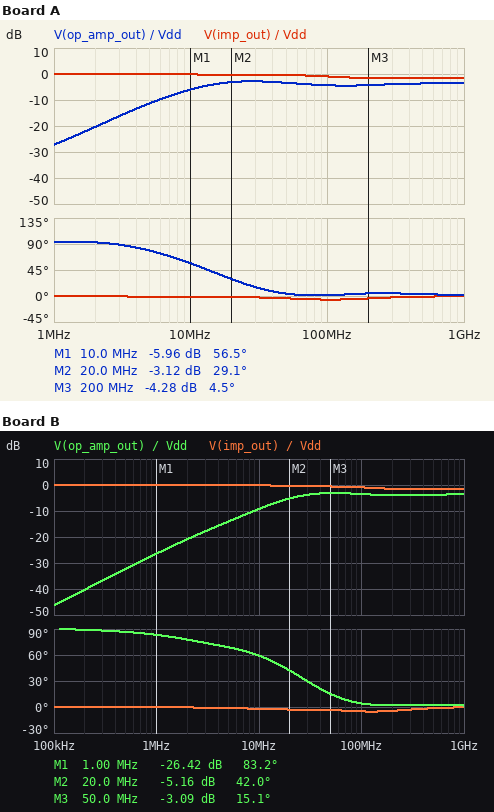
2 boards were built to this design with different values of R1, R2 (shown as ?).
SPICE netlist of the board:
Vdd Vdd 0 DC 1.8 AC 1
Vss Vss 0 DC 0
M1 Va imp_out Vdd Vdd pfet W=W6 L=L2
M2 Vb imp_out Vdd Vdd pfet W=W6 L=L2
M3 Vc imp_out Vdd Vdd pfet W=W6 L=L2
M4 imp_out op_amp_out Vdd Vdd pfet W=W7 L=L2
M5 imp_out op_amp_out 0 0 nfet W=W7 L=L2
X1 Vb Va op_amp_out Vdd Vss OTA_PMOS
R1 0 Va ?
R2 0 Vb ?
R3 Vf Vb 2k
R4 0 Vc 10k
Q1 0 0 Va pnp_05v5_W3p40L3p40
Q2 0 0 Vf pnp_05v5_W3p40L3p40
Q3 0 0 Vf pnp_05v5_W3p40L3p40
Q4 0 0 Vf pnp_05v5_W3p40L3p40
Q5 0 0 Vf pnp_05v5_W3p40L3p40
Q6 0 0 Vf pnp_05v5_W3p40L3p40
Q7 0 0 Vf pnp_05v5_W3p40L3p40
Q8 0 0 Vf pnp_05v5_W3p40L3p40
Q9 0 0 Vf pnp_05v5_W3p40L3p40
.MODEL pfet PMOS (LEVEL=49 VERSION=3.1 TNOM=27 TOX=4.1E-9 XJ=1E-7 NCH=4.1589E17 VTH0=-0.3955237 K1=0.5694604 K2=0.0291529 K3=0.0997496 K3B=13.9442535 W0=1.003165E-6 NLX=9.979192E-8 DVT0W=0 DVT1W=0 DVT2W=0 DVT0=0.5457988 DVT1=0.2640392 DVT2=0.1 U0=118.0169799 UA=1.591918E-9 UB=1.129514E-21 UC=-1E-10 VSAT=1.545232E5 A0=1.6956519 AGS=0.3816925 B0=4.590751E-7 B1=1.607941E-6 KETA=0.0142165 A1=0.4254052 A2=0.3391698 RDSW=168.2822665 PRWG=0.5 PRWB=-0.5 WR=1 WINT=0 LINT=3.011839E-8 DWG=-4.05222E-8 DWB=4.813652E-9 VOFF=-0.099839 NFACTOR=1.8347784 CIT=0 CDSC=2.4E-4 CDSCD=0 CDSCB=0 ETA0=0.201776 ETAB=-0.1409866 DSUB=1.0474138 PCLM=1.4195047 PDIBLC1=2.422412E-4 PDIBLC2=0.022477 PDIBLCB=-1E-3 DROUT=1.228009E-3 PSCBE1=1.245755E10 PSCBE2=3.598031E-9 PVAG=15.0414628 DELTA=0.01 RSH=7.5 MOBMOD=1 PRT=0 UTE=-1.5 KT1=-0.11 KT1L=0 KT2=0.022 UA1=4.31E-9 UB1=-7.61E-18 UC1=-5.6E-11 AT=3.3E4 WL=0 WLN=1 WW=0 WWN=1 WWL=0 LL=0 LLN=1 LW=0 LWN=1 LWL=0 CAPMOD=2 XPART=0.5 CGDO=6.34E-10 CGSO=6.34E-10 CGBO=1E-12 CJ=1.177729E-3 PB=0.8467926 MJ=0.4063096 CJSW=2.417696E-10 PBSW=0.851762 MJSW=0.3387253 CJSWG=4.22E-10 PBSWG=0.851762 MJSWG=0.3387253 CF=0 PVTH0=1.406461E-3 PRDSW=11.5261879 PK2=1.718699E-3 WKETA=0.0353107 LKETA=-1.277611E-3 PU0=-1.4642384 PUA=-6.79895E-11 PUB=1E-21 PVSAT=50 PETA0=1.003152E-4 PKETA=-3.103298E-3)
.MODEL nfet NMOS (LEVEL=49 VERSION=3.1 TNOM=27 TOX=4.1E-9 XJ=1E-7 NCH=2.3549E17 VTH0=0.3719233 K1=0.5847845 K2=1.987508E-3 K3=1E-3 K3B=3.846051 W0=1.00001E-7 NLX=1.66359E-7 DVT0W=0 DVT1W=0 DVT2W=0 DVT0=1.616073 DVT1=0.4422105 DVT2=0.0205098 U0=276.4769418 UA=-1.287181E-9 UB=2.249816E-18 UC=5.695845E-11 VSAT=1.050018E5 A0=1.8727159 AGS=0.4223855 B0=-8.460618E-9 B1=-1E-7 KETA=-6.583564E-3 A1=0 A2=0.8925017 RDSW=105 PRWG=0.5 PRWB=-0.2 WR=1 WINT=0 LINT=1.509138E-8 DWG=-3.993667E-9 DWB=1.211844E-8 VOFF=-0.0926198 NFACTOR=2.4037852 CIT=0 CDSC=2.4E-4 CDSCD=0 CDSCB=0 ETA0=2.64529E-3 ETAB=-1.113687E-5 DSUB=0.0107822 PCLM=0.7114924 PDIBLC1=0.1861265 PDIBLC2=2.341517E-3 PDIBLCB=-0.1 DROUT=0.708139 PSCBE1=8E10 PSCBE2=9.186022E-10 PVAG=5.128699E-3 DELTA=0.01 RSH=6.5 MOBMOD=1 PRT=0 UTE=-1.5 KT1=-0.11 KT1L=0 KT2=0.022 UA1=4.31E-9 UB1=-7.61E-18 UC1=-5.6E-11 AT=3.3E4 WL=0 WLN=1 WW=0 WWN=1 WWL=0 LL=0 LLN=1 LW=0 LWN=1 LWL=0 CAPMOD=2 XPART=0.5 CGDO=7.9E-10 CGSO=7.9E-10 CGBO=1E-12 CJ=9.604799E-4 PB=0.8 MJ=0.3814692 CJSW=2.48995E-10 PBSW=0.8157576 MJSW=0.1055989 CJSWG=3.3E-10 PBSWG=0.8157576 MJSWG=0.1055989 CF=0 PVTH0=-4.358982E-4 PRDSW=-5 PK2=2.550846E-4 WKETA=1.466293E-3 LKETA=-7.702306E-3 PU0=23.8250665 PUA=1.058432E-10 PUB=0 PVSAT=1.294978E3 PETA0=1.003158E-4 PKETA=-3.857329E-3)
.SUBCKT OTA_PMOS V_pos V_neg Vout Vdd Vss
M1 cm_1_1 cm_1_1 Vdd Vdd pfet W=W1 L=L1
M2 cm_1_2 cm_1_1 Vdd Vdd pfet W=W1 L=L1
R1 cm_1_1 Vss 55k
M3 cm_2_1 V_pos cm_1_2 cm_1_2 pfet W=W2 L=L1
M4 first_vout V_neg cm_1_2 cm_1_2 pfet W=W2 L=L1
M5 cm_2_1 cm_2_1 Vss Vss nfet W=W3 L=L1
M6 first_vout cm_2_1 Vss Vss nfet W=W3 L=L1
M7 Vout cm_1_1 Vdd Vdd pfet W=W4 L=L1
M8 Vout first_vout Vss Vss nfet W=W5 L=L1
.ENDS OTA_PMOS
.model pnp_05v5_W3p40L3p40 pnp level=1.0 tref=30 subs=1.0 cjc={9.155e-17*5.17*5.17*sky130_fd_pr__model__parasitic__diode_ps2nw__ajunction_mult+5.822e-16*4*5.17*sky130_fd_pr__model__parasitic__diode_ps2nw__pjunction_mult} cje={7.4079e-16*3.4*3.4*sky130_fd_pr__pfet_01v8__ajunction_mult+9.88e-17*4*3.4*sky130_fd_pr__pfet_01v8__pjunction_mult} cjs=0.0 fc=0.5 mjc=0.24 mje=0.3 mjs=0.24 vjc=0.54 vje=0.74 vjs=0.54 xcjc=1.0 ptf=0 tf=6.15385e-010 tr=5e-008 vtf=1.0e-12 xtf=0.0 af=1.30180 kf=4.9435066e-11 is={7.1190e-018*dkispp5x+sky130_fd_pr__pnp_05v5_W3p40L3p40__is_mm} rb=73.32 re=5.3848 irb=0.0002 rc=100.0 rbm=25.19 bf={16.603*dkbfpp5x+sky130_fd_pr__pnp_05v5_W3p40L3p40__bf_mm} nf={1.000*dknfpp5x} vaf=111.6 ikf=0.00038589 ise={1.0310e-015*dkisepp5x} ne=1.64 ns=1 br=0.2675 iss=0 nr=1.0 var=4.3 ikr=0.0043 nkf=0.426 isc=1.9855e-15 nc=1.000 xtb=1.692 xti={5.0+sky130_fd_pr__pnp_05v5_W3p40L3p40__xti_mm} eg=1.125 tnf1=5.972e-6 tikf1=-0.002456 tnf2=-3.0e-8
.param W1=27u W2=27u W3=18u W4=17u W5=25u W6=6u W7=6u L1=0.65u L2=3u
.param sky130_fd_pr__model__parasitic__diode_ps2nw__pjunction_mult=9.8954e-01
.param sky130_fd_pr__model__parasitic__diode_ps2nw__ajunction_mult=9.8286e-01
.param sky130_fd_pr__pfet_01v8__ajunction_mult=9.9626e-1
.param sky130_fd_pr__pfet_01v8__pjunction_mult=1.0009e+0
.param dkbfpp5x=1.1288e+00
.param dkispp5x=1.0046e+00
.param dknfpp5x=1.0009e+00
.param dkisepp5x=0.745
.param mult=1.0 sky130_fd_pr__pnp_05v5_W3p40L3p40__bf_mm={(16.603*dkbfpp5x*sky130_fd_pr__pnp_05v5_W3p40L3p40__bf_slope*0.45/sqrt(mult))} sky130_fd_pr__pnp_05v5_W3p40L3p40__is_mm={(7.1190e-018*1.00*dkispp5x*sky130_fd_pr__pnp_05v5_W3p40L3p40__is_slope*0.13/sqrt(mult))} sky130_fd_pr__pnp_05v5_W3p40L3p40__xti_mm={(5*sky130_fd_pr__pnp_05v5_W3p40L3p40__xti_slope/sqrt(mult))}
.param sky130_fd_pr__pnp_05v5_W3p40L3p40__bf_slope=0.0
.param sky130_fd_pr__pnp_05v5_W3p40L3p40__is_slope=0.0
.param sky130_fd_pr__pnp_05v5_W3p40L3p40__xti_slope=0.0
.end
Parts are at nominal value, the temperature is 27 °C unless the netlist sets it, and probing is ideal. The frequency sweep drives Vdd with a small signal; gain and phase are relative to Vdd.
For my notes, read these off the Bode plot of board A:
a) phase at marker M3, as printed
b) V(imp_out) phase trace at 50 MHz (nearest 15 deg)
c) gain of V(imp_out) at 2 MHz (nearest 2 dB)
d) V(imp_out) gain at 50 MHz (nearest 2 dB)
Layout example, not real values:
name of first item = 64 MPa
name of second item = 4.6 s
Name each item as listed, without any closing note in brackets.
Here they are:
phase at marker M3, as printed = 4.5 deg
V(imp_out) phase trace at 50 MHz = 0 deg
gain of V(imp_out) at 2 MHz = 0 dB
V(imp_out) gain at 50 MHz = 0 dB
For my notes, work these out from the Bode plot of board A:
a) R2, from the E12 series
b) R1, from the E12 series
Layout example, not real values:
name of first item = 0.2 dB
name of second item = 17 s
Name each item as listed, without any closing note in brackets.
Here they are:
R2, from the E12 series = 56 kΩ
R1, from the E12 series = 22 kΩ
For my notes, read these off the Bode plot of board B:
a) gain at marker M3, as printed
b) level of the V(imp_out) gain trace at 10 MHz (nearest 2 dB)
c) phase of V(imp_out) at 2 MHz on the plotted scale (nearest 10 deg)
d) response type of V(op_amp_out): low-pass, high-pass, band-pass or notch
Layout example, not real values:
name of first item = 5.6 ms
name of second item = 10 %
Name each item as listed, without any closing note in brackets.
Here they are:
gain at marker M3, as printed = -3.09 dB
level of the V(imp_out) gain trace at 10 MHz = 0 dB
phase of V(imp_out) at 2 MHz on the plotted scale = 0 deg
response type of V(op_amp_out): low-pass, high-pass, band-pass or notch = high-pass
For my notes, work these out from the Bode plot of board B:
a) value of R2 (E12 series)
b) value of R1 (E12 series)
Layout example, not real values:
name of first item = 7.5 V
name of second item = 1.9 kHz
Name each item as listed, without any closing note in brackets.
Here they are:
value of R2 = 39 kΩ
value of R1 = 6.8 kΩ
